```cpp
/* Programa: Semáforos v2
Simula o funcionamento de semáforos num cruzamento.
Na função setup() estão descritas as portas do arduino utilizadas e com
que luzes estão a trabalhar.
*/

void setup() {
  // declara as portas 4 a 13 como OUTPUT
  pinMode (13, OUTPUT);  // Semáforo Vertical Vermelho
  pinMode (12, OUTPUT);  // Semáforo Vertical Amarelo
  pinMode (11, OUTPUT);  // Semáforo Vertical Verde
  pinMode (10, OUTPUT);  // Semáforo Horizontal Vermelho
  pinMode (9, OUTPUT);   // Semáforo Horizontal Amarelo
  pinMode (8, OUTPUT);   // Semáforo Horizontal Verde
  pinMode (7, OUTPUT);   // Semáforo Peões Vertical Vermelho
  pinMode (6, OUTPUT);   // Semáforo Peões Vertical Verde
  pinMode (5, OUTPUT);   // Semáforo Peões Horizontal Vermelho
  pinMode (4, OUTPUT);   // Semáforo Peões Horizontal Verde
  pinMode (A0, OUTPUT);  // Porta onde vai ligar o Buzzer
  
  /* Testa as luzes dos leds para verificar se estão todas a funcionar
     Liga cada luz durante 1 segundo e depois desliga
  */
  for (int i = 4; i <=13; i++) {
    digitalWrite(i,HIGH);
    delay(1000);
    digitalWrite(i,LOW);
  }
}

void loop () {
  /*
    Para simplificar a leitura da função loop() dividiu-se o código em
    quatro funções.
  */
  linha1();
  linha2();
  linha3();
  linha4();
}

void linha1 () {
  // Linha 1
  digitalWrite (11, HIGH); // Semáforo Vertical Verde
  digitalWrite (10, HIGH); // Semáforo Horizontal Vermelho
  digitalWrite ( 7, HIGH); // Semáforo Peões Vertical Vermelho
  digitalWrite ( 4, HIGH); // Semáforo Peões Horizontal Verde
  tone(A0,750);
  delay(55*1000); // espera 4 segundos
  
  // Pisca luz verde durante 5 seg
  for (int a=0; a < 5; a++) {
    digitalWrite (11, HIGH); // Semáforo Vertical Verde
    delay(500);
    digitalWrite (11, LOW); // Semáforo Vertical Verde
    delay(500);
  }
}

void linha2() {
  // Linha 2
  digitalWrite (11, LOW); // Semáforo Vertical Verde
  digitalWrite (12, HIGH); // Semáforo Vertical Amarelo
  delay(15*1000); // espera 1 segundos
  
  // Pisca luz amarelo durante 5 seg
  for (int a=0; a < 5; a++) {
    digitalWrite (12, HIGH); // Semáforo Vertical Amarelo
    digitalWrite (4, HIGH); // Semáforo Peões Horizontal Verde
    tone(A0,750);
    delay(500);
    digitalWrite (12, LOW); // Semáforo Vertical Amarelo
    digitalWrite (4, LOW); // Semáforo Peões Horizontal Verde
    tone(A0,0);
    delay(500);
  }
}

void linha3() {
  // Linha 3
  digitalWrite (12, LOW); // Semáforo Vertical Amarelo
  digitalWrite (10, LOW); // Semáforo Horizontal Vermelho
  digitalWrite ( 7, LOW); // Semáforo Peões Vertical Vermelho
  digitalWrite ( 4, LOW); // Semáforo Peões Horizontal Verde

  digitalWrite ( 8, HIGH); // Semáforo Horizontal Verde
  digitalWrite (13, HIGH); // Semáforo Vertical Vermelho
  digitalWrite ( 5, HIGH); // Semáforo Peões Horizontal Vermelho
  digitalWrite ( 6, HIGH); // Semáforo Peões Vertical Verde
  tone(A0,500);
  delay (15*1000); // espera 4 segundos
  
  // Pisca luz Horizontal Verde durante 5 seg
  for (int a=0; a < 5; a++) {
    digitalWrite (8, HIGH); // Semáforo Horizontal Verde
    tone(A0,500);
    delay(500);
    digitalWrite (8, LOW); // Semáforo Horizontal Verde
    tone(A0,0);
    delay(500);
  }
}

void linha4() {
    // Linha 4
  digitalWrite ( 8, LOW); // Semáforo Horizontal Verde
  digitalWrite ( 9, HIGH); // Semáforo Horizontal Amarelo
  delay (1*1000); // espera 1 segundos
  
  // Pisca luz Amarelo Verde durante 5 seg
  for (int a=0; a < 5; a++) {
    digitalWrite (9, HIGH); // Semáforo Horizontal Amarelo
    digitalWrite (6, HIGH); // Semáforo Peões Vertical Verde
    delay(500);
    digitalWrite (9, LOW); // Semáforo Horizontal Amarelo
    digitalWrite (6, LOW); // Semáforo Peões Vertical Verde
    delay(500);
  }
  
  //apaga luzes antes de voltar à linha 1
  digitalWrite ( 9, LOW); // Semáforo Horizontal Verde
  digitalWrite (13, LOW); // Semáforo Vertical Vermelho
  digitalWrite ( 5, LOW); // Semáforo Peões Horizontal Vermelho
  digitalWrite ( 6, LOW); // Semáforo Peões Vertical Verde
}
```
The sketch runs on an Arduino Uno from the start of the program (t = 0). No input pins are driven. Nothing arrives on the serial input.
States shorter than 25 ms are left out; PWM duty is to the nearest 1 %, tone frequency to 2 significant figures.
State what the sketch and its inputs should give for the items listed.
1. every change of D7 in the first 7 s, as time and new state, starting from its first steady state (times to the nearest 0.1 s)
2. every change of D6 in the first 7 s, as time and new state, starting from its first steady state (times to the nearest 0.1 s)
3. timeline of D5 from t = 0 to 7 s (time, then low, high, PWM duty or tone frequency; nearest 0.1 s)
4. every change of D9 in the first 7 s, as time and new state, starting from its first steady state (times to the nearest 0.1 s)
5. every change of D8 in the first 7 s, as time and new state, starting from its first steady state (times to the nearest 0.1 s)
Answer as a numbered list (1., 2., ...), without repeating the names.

1. 0 s low; 3 s high; 4 s low
2. 0 s low; 2 s high; 3 s low
3. 0 s low; 1 s high; 2 s low
4. 0 s low; 5 s high; 6 s low
5. 0 s low; 4 s high; 5 s low
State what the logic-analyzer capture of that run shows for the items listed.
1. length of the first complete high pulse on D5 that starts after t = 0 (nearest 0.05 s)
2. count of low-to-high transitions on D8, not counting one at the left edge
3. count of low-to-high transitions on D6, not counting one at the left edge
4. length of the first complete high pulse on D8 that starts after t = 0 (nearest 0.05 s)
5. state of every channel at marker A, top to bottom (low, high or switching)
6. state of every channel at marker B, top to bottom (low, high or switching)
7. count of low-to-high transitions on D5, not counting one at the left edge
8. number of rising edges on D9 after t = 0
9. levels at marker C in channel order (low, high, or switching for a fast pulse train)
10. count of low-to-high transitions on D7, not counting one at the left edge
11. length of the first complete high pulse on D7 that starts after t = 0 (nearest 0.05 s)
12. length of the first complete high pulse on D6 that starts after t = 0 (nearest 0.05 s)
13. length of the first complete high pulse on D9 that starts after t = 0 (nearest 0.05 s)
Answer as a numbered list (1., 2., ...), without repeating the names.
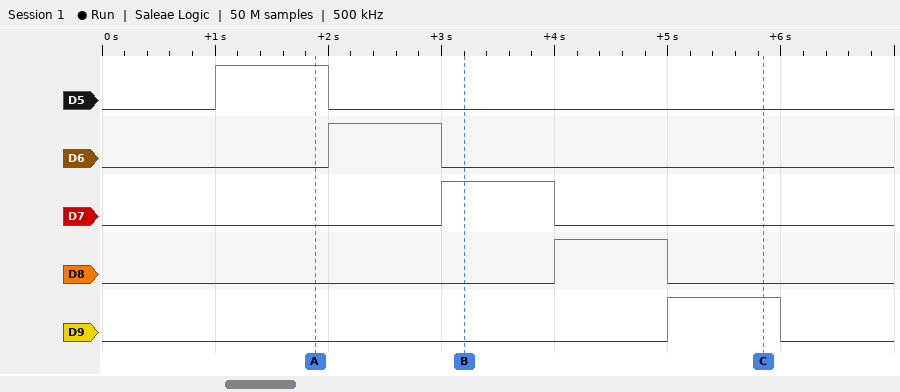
1. 1.00 s
2. 1
3. 1
4. 1.00 s
5. D5 high, D6 low, D7 low, D8 low, D9 low
6. D5 low, D6 low, D7 high, D8 low, D9 low
7. 1
8. 1
9. D5 low, D6 low, D7 low, D8 low, D9 high
10. 1
11. 1.00 s
12. 1.00 s
13. 1.00 s
